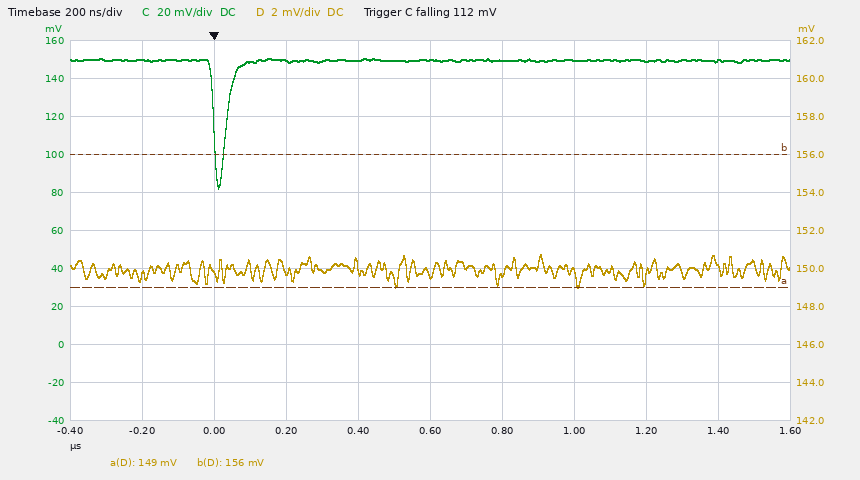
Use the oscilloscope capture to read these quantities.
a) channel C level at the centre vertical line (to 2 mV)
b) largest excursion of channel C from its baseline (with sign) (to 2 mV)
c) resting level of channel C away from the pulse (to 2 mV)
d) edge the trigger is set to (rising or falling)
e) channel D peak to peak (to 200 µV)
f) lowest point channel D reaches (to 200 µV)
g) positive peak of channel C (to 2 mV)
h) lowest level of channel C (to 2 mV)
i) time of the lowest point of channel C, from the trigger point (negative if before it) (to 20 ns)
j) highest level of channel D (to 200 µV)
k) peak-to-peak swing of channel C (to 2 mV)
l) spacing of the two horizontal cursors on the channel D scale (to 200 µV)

150 mV
-68 mV
150 mV
falling
1.8 mV
149.0 mV
150 mV
82 mV
+20 ns
150.8 mV
68 mV
7.0 mV
